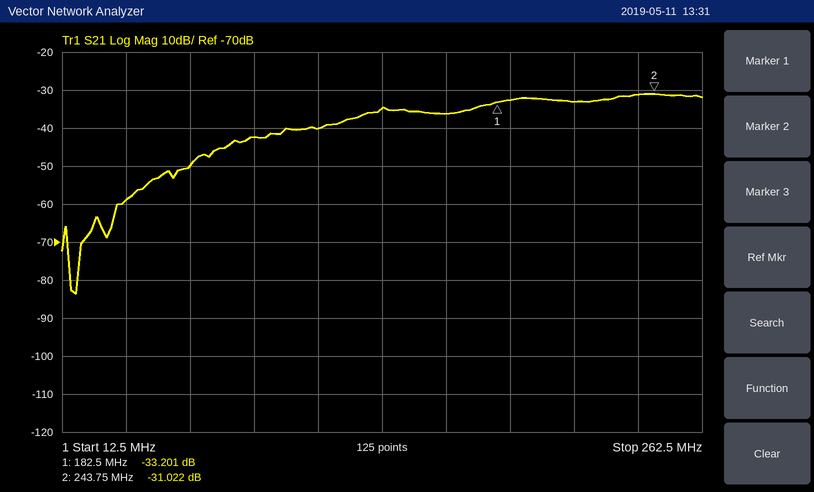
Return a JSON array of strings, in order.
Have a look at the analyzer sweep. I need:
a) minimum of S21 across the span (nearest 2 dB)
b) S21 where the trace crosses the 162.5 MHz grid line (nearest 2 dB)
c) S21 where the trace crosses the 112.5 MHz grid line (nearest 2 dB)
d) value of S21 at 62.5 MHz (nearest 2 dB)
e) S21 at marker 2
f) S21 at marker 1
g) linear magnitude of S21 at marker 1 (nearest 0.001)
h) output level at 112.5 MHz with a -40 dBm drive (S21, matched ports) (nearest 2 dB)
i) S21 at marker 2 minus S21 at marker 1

["-84 dB", "-36 dB", "-40 dB", "-50 dB", "-31.022 dB", "-33.201 dB", "0.022", "-80 dBm", "2.179 dB"]
